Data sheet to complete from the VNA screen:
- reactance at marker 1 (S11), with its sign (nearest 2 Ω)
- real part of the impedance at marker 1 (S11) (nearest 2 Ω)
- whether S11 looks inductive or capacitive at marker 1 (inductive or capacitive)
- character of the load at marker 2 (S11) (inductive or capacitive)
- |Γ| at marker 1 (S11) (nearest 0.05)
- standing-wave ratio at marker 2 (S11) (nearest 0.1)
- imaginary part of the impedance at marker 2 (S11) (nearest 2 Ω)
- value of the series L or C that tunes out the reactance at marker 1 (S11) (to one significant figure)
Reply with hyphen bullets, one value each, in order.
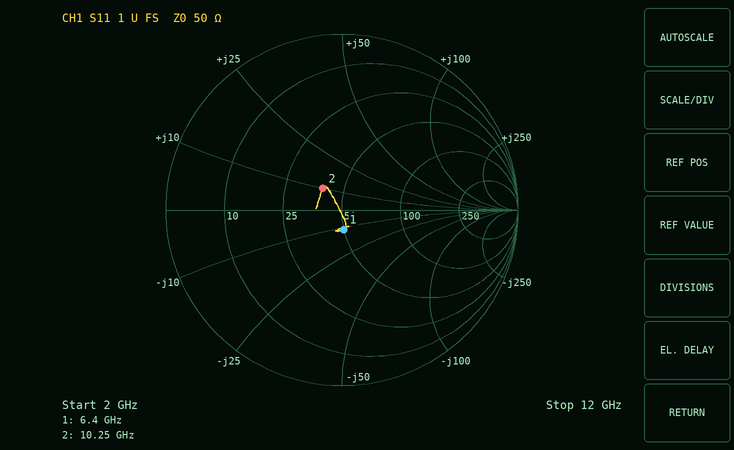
- -12 Ω
- 50 Ω
- capacitive
- inductive
- 0.10
- 1.4
- +10 Ω
- 300 pH
